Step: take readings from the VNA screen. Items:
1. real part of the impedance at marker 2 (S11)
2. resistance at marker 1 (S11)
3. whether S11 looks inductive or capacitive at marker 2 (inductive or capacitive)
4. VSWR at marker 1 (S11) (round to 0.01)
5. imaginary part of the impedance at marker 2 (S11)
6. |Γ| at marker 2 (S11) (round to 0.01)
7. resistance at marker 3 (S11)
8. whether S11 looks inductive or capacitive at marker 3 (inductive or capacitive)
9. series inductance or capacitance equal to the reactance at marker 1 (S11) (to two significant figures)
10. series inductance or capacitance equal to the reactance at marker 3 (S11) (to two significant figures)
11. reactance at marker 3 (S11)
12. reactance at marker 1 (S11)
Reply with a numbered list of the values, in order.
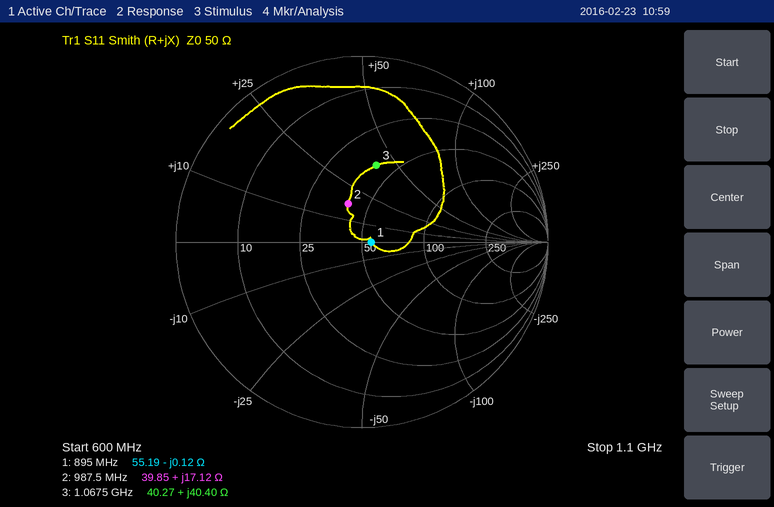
1. 39.85 Ω
2. 55.19 Ω
3. inductive
4. 1.10
5. +17.12 Ω
6. 0.22
7. 40.27 Ω
8. inductive
9. 1.5 nF
10. 6.0 nH
11. +40.40 Ω
12. -0.12 Ω
